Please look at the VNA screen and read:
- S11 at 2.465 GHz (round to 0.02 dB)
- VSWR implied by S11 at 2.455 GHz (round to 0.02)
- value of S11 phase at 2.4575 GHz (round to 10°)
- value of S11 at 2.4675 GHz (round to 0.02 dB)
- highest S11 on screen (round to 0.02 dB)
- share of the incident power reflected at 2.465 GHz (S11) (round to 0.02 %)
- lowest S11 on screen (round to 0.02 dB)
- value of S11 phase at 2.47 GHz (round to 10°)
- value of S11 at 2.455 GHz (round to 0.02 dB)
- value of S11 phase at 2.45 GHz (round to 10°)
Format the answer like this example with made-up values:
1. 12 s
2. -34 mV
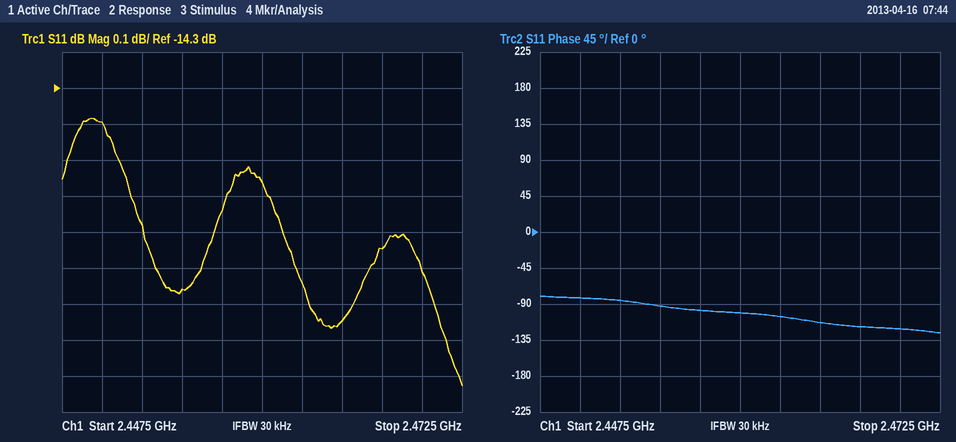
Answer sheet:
1. -14.94 dB
2. 1.44
3. -100°
4. -14.74 dB
5. -14.38 dB
6. 3.20 %
7. -15.12 dB
8. -120°
9. -14.86 dB
10. -80°
